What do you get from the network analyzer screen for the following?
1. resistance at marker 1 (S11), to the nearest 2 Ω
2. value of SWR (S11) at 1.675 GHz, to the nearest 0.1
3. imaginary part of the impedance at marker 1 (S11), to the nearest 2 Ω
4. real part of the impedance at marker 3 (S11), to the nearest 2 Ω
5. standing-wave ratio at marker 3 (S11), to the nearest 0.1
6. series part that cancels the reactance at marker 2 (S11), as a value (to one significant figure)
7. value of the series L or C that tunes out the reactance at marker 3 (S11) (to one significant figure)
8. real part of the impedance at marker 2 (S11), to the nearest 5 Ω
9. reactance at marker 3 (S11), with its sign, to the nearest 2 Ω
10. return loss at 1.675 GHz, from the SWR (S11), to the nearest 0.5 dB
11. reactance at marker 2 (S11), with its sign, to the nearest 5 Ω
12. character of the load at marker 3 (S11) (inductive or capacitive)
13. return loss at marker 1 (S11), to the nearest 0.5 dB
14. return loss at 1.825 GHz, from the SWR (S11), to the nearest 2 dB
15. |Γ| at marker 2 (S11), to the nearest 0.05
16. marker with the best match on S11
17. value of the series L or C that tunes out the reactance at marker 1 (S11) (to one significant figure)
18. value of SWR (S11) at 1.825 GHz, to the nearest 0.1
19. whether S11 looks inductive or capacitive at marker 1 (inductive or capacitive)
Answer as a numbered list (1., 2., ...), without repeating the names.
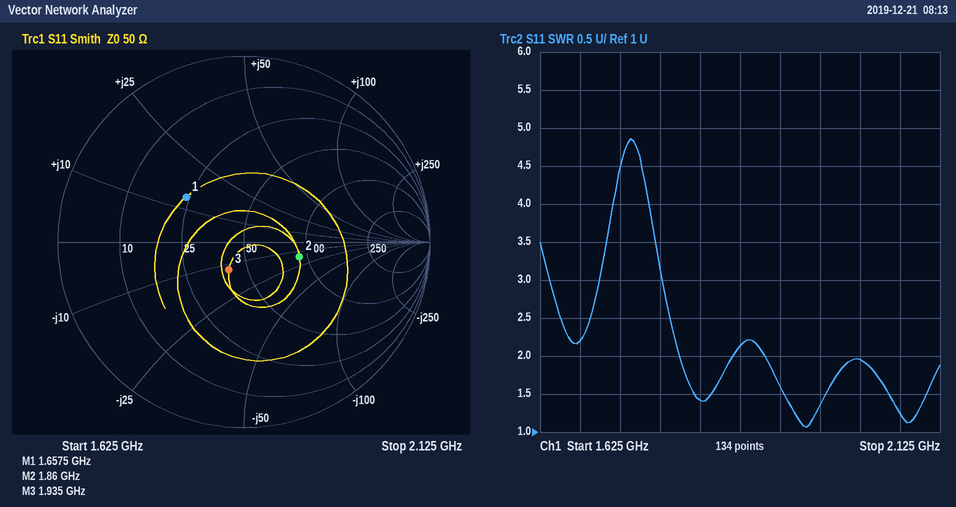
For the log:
1. 24 Ω
2. 2.2
3. +14 Ω
4. 40 Ω
5. 1.4
6. 1 nH
7. 1 nH
8. 90 Ω
9. -12 Ω
10. 8.5 dB
11. -15 Ω
12. capacitive
13. 8.0 dB
14. 16 dB
15. 0.30
16. marker 3
17. 7 pF
18. 1.4
19. inductive
